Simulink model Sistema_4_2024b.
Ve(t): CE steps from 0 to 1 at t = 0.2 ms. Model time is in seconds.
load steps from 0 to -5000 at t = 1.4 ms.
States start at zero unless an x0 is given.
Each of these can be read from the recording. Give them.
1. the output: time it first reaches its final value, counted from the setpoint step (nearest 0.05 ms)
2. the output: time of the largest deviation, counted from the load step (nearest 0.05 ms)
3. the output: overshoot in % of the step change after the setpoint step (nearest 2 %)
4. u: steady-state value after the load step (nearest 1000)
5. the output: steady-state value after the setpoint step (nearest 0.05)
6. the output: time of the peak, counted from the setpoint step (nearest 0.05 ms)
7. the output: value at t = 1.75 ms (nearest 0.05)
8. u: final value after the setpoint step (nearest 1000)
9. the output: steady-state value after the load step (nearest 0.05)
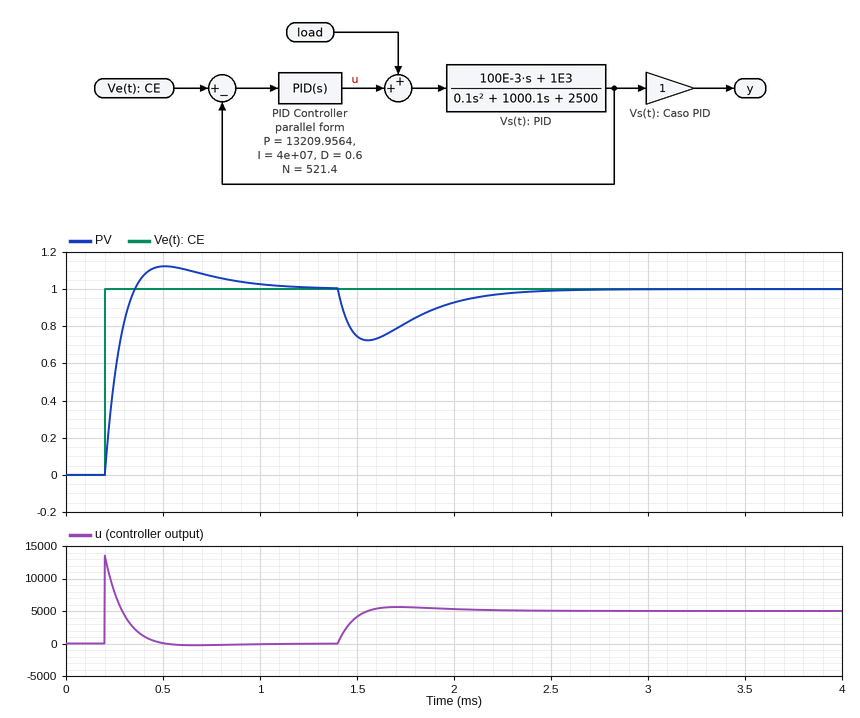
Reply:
0.15 ms
0.15 ms
12 %
5000
1.00
0.30 ms
0.80
0
1.00
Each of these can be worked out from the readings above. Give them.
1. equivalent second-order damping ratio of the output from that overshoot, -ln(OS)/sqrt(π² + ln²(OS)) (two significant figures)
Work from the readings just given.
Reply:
0.56
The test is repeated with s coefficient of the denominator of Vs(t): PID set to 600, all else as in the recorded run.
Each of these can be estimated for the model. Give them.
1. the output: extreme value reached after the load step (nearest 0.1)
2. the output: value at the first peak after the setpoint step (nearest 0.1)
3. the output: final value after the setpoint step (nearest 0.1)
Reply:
0.7
1.2
1.0
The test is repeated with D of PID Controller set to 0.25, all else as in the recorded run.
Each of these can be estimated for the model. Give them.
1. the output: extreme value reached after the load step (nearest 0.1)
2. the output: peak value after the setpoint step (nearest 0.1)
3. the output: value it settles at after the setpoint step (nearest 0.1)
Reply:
0.7
1.1
1.0
